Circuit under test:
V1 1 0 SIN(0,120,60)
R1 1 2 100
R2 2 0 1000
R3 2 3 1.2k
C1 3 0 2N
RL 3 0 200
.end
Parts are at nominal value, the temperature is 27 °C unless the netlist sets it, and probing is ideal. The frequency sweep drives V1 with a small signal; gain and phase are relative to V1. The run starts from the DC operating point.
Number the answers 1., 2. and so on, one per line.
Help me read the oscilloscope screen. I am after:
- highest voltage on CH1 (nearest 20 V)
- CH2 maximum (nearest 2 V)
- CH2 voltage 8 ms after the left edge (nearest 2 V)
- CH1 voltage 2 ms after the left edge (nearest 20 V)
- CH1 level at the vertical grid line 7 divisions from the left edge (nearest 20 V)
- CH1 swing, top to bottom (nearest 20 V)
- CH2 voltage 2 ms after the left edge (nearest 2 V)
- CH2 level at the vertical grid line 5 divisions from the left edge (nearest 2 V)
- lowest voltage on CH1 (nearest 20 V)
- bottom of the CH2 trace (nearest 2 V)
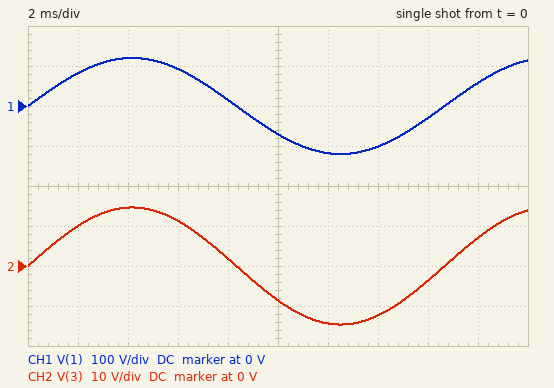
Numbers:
1. 120 V
2. 14 V
3. 2 V
4. 80 V
5. -100 V
6. 240 V
7. 10 V
8. -8 V
9. -120 V
10. -14 V
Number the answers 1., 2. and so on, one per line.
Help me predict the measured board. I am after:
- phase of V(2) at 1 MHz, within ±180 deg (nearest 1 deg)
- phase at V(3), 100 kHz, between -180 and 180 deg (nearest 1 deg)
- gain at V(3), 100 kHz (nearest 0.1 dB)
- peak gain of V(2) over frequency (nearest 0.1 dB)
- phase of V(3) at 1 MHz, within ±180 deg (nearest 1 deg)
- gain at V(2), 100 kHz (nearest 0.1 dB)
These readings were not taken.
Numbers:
1. 0 deg
2. -12 deg
3. -18.5 dB
4. -1.4 dB
5. -65 deg
6. -1.4 dB
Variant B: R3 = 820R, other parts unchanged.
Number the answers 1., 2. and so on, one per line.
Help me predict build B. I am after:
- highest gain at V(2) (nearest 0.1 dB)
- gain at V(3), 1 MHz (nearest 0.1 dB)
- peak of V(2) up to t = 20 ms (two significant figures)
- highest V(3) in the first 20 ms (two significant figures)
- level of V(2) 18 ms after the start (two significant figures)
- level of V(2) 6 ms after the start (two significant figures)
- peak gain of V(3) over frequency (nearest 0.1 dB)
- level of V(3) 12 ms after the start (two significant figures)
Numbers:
1. -1.6 dB
2. -22.9 dB
3. 100 V
4. 20 V
5. 48 V
6. 77 V
7. -15.7 dB
8. -19 V
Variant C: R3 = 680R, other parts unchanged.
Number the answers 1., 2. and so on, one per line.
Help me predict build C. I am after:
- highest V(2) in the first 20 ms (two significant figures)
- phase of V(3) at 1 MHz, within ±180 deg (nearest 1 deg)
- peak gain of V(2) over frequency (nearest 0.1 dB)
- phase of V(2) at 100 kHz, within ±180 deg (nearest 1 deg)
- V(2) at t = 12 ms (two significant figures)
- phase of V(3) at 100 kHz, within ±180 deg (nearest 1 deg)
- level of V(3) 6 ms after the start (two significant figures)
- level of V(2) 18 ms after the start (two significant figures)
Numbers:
1. 99 V
2. -63 deg
3. -1.7 dB
4. 0 deg
5. -97 V
6. -11 deg
7. 17 V
8. 48 V
